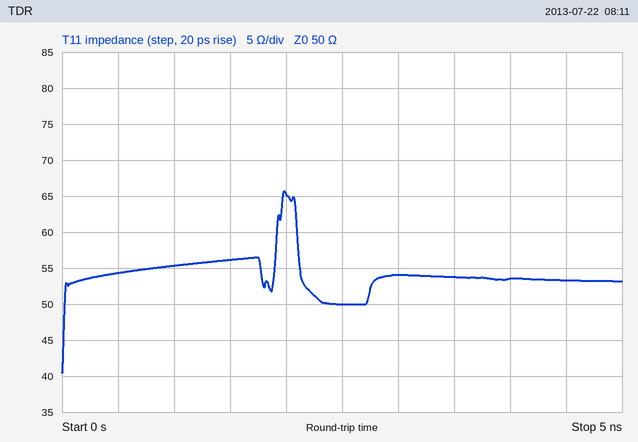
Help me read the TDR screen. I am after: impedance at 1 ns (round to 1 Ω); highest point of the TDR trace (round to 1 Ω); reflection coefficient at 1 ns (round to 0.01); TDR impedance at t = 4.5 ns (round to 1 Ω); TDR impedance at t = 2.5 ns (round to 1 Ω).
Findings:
55 Ω
66 Ω
+0.05
53 Ω
50 Ω
